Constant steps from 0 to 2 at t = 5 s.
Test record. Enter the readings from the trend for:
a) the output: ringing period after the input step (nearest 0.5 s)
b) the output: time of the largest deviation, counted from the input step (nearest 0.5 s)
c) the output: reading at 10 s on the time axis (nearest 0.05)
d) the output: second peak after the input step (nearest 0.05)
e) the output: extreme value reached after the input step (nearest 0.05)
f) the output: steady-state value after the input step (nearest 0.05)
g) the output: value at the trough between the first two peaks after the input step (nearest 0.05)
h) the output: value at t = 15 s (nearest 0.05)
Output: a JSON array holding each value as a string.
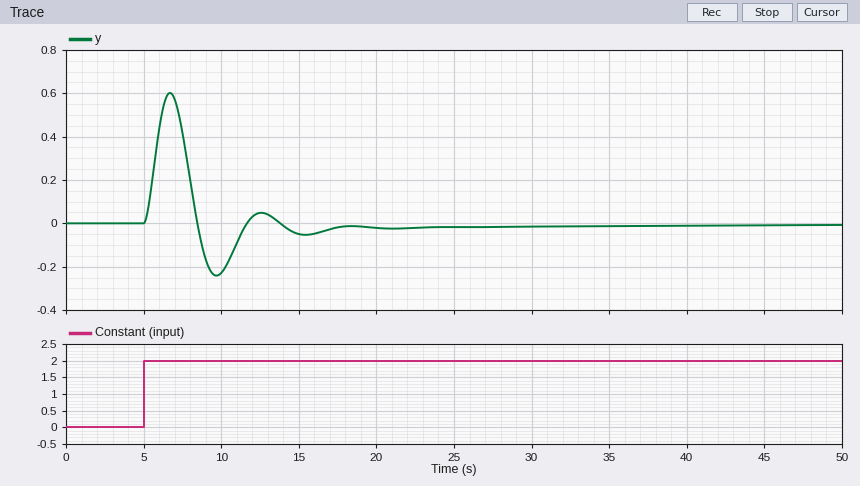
["6.0 s", "1.5 s", "-0.25", "0.05", "0.60", "0.00", "-0.25", "-0.05"]
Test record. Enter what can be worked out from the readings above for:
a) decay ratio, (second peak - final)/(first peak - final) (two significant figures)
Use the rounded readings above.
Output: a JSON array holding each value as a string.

["0.083"]
